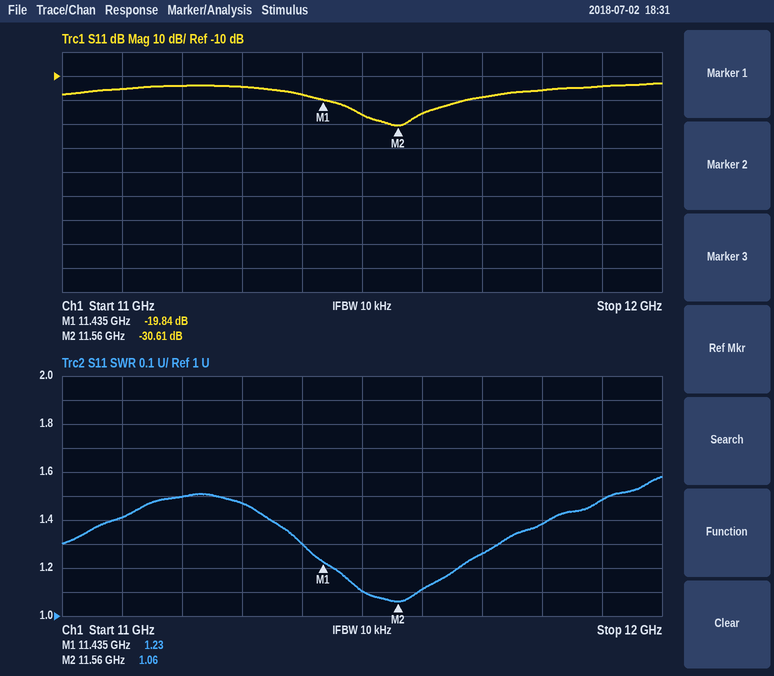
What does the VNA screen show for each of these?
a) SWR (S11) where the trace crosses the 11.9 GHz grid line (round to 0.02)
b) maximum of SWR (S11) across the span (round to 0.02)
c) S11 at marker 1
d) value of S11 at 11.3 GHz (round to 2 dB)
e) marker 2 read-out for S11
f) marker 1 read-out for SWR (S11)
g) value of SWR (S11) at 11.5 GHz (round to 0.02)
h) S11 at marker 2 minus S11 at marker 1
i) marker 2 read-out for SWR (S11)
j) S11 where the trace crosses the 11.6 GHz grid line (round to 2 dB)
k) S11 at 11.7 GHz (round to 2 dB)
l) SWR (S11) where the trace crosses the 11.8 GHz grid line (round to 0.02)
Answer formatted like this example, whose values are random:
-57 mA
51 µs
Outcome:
1.48
1.58
-19.84 dB
-14 dB
-30.61 dB
1.23
1.10
-10.77 dB
1.06
-26 dB
-18 dB
1.38
